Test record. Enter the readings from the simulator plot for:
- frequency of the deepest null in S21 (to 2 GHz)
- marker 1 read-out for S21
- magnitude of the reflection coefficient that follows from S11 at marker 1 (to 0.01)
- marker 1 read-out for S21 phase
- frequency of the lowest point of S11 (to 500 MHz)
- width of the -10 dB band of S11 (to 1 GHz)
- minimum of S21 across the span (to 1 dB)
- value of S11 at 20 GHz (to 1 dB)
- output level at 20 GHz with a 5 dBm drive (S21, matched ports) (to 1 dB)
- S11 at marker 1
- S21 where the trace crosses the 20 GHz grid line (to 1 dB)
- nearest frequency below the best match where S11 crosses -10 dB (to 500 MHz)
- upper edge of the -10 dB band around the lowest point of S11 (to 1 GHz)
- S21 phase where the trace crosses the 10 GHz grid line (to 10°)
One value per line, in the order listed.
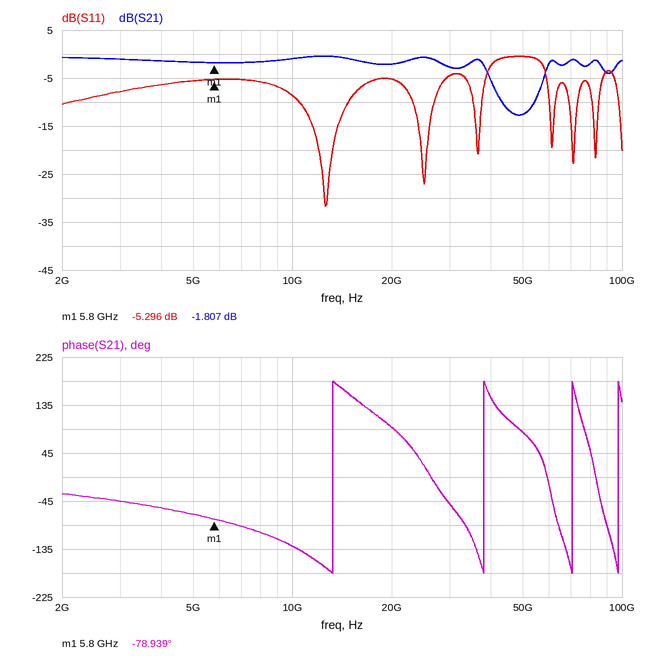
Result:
48 GHz
-1.807 dB
0.54
-78.939°
12.5 GHz
4 GHz
-13 dB
-5 dB
3 dBm
-5.296 dB
-2 dB
10.5 GHz
15 GHz
-130°
